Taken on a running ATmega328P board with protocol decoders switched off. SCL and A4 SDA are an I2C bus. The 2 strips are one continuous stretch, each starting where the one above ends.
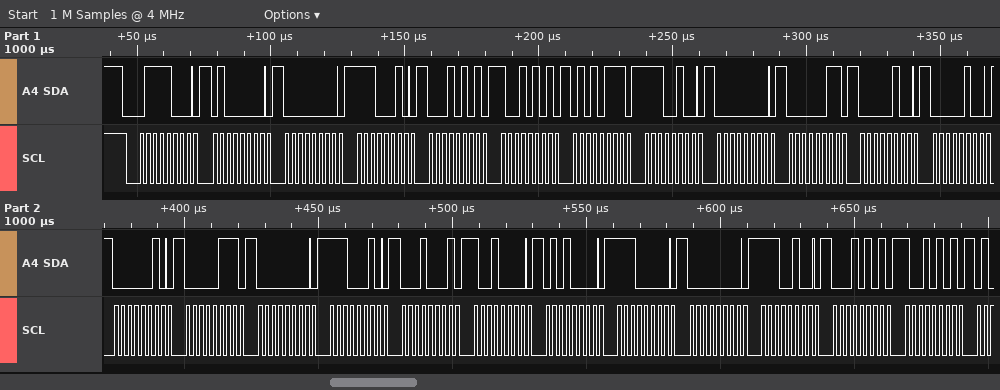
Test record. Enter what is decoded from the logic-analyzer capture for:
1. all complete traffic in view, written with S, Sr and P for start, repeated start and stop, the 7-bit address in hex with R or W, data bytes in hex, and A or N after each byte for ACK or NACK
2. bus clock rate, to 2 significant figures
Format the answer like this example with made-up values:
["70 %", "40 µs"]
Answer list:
["S 3CW A 40 A 00 A E2 A 15 A 95 A 57 A E4 A 00 A 03 A 04 A 04 A 02 A 07 A 00 A E2 A 11 A 90 A 50 A E0 A 00 A E4 A 15 A 95 A", "400 kHz"]
